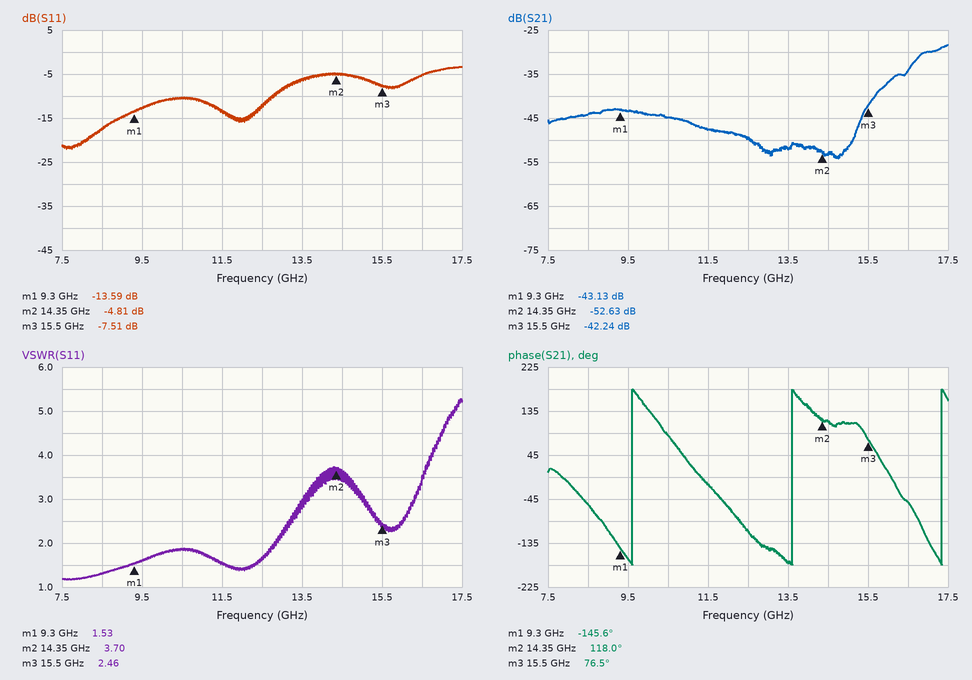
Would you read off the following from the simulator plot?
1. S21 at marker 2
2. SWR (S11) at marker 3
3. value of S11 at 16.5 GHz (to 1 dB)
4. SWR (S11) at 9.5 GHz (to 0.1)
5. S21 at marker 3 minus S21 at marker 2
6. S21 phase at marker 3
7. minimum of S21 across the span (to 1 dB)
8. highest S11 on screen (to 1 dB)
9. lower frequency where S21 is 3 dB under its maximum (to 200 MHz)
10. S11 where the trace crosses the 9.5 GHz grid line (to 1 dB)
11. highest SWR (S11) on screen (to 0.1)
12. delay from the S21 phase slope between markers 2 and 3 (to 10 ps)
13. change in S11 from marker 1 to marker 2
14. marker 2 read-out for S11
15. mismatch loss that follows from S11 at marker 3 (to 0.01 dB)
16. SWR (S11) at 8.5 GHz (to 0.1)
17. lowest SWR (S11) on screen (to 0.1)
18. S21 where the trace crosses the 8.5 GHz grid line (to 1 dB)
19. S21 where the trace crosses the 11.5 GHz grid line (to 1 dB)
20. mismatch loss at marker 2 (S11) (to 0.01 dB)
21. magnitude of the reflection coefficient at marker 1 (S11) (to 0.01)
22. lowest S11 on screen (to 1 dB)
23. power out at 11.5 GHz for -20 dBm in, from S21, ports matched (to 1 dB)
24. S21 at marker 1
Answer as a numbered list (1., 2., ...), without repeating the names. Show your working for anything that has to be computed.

1. -52.63 dB
2. 2.46
3. -5 dB
4. 1.6
5. -42.24 − (-52.63) = 10.39 dB
6. 76.5°
7. -54 dB
8. -3 dB
9. 16.8 GHz
10. -13 dB
11. 5.3
12. −(76.5° − (118°))/(360° × 1.15 GHz) ≈ 100 ps
13. -4.81 − (-13.59) = 8.78 dB
14. -4.81 dB
15. −10 log10(1 − 10^(-7.51/10)) ≈ 0.85 dB
16. 1.3
17. 1.2
18. -44 dB
19. -48 dB
20. −10 log10(1 − 10^(-4.81/10)) ≈ 1.74 dB
21. 10^(-13.59/20) ≈ 0.21
22. -22 dB
23. -20 dBm + (-48 dB) = -68 dBm
24. -43.13 dB
